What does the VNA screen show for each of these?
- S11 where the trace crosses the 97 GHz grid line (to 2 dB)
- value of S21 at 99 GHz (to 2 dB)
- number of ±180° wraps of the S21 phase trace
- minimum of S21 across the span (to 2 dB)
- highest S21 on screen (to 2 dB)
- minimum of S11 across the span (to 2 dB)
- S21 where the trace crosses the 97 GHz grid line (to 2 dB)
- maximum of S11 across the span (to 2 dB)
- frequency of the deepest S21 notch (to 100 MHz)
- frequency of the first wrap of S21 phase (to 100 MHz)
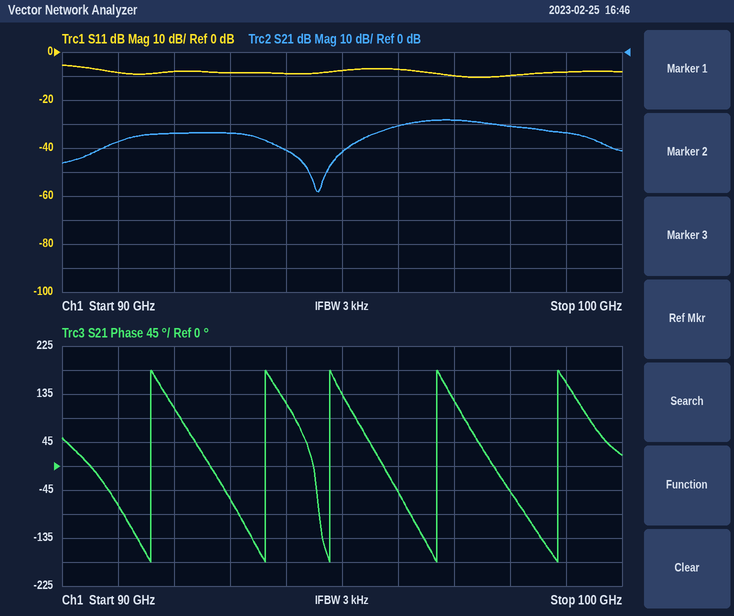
-10 dB
-34 dB
5
-58 dB
-28 dB
-10 dB
-28 dB
-6 dB
94.6 GHz
91.6 GHz
